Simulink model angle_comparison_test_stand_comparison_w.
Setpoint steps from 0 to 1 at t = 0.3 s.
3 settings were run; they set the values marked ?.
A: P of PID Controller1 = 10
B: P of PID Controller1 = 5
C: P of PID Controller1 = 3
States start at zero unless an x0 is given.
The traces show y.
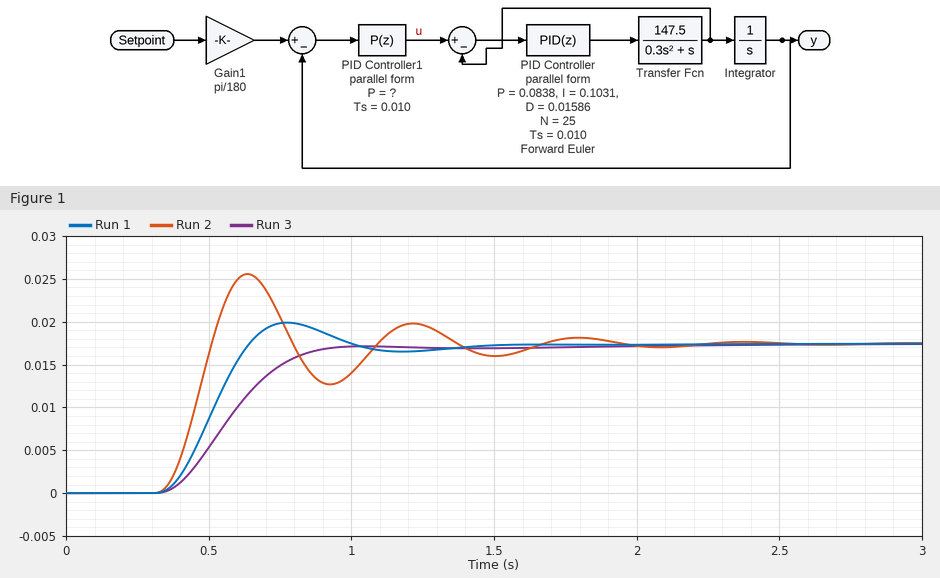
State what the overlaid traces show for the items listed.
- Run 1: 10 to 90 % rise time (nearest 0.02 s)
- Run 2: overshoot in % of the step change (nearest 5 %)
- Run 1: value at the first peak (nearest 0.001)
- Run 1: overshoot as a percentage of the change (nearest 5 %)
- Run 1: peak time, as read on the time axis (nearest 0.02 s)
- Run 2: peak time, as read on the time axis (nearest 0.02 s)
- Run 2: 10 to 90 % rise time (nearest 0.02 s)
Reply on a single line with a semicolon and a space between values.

0.22 s; 45 %; 0.020; 15 %; 0.78 s; 0.64 s; 0.12 s
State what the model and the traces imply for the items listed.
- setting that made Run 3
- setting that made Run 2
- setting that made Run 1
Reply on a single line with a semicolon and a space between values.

C; A; B
